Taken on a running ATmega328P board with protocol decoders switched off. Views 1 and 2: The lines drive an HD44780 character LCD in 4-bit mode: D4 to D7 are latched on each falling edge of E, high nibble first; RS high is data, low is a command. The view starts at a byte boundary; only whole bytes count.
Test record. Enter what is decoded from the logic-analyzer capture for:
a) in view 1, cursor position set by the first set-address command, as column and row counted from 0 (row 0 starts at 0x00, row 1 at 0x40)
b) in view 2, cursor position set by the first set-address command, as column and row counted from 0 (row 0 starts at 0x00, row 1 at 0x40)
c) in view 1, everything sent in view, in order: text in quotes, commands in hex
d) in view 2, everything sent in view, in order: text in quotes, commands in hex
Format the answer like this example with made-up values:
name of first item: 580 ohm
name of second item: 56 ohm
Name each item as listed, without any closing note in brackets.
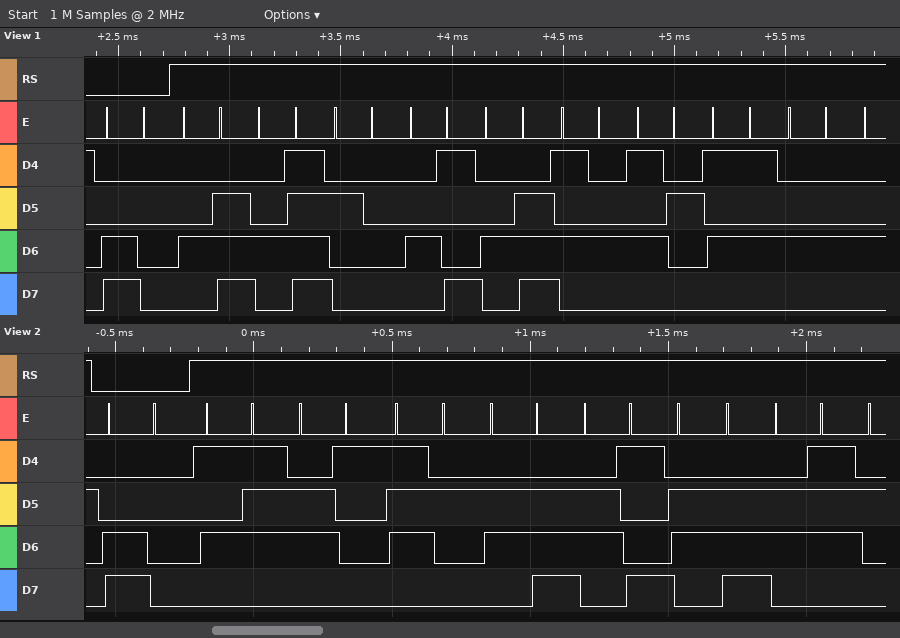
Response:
in view 1, cursor position set by the first set-address command, as column and row counted from 0: column 0, row 1
in view 2, cursor position set by the first set-address command, as column and row counted from 0: column 0, row 1
in view 1, everything sent in view, in order: text in quotes, commands in hex: 0xC0 "NO INTRUD"
in view 2, everything sent in view, in order: text in quotes, commands in hex: 0xC0 "Warning"
